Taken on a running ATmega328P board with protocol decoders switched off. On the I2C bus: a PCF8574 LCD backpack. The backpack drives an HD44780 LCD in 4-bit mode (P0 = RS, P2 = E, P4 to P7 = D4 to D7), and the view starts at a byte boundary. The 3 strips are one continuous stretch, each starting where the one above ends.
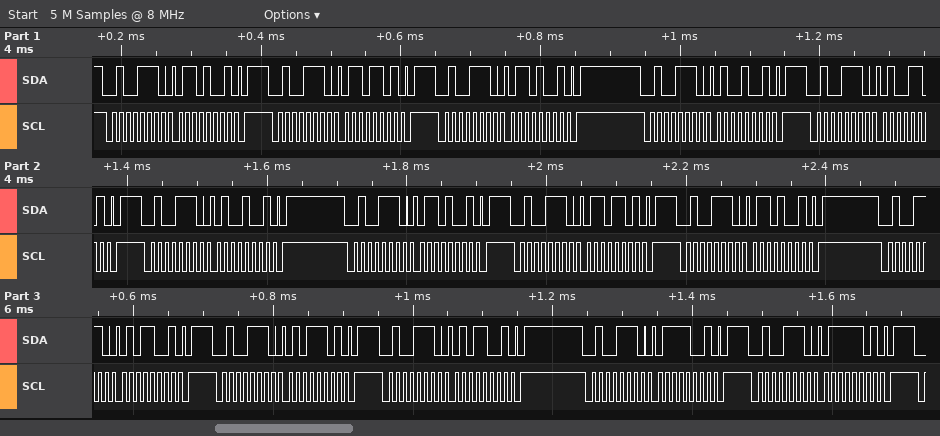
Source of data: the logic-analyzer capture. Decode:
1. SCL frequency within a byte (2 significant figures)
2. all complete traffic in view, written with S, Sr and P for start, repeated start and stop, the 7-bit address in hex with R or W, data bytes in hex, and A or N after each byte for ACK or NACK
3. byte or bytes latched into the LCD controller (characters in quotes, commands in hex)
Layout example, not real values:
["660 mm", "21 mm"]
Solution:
["100 kHz", "S 27W A 69 A P S 27W A 6D A P S 27W A 69 A P S 27W A 49 A P S 27W A 4D A P S 27W A 49 A P S 27W A 69 A P S 27W A 6D A P S 27W A 69 A P S 27W A 59 A P S 27W A 5D A P S 27W A 59 A P S 27W A 79 A P S 27W A 7D A P", "'d' 'e'"]
